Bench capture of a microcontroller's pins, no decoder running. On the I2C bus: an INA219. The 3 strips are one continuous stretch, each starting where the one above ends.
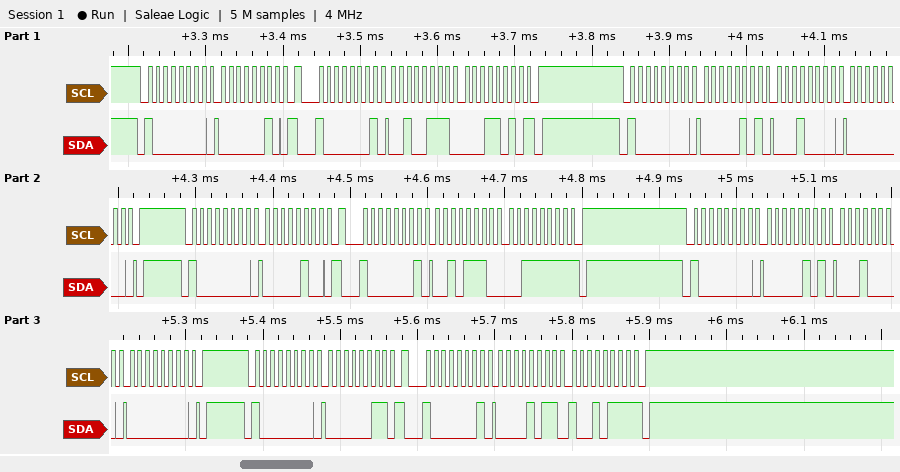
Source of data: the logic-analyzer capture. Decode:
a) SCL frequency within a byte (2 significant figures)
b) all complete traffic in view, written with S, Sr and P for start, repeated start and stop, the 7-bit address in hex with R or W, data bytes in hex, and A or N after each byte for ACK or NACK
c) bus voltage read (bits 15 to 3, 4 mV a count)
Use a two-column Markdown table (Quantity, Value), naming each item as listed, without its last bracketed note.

| Quantity | Value |
|---|---|
| SCL frequency within a byte | 100 kHz |
| all complete traffic in view, written with S, Sr and P for start, repeated start and stop, the 7-bit address in hex with R or W, data bytes in hex, and A or N after each byte for ACK or NACK | S 40W A 02 A Sr 40R A 27 A 1A N P S 40W A 05 A 10 A 00 A P S 40W A 04 A Sr 40R A 2E A 3F N P S 40W A 05 A 10 A 00 A P S 40W A 03 A Sr 40R A 0B A 97 N P |
| bus voltage read | 5.004 V |
